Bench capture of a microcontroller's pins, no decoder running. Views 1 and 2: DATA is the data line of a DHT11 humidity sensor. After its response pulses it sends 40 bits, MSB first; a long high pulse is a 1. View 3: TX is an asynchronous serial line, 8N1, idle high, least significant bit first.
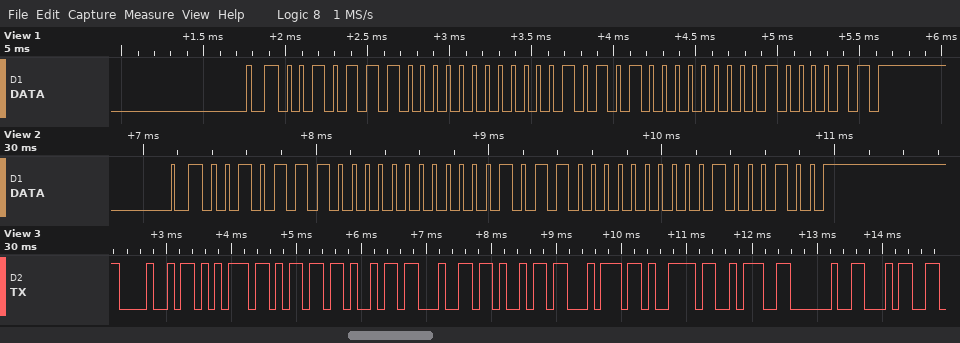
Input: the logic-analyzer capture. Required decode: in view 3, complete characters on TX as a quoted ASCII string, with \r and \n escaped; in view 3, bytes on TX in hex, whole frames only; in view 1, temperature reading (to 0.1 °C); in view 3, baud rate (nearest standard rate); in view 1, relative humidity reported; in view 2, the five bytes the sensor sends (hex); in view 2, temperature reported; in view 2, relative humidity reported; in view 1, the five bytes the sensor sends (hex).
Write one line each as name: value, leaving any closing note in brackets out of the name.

in view 3, complete characters on TX as a quoted ASCII string, with \r and \n escaped: "Humidity: 4"
in view 3, bytes on TX in hex, whole frames only: 0x48 0x75 0x6D 0x69 0x64 0x69 0x74 0x79 0x3A 0x20 0x34
in view 1, temperature reading: 21.0 °C
in view 3, baud rate: 9600 baud
in view 1, relative humidity reported: 46 %
in view 2, the five bytes the sensor sends: 2E 00 16 00 44
in view 2, temperature reported: 22.0 °C
in view 2, relative humidity reported: 46 %
in view 1, the five bytes the sensor sends: 2E 00 15 00 43
